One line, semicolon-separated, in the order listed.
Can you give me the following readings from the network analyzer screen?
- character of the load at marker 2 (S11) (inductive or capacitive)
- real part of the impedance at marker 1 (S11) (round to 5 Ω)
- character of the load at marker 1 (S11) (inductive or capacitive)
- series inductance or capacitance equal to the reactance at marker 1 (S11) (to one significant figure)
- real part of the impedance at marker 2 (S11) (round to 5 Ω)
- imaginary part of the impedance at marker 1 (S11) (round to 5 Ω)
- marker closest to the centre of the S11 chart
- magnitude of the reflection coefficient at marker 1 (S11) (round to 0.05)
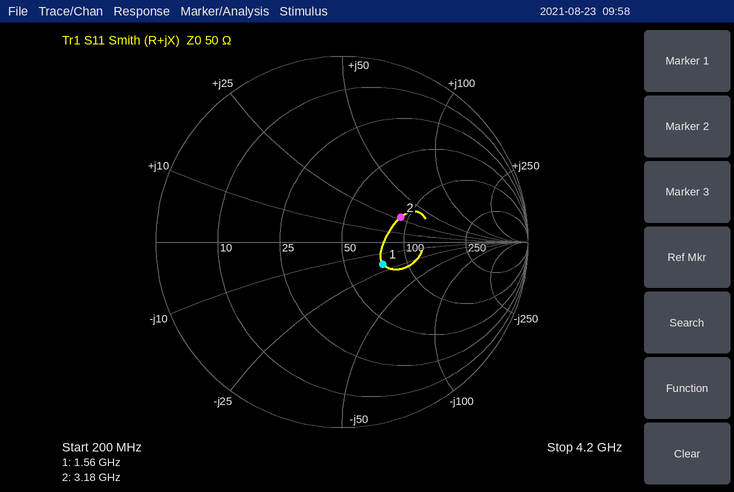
inductive; 75 Ω; capacitive; 5 pF; 90 Ω; -20 Ω; marker 1; 0.25
